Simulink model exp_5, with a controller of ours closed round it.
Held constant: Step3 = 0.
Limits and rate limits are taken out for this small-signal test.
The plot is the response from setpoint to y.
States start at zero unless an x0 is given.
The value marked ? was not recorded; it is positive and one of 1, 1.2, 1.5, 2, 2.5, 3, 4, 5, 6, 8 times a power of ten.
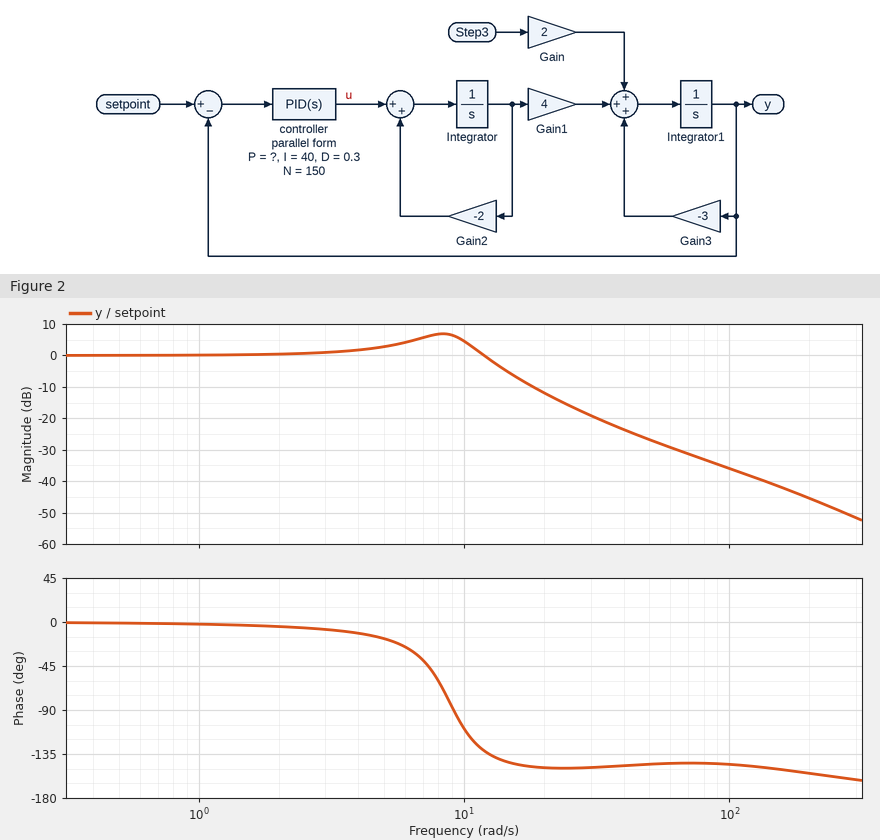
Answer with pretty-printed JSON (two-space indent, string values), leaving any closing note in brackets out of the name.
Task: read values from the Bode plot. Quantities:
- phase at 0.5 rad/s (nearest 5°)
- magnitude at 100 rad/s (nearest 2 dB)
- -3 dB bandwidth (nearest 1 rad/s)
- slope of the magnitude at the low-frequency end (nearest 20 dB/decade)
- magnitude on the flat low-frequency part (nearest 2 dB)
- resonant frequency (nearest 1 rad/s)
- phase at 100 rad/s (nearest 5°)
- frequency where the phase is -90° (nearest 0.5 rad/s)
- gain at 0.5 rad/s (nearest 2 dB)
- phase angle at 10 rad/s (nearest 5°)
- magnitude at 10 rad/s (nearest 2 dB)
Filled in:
{
  "phase at 0.5 rad/s": "0°",
  "magnitude at 100 rad/s": "-36 dB",
  "-3 dB bandwidth": "13 rad/s",
  "slope of the magnitude at the low-frequency end": "0 dB/decade",
  "magnitude on the flat low-frequency part": "0 dB",
  "resonant frequency": "8 rad/s",
  "phase at 100 rad/s": "-145°",
  "frequency where the phase is -90°": "9.0 rad/s",
  "gain at 0.5 rad/s": "0 dB",
  "phase angle at 10 rad/s": "-110°",
  "magnitude at 10 rad/s": "4 dB"
}
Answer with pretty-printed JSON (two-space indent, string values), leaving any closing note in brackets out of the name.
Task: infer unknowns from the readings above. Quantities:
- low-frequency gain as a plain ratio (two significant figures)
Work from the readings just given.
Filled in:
{
  "low-frequency gain as a plain ratio": "1.0"
}
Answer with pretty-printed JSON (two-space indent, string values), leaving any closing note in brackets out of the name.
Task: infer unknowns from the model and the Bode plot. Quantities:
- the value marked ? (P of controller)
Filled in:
{
  "the value marked ?": "20"
}
